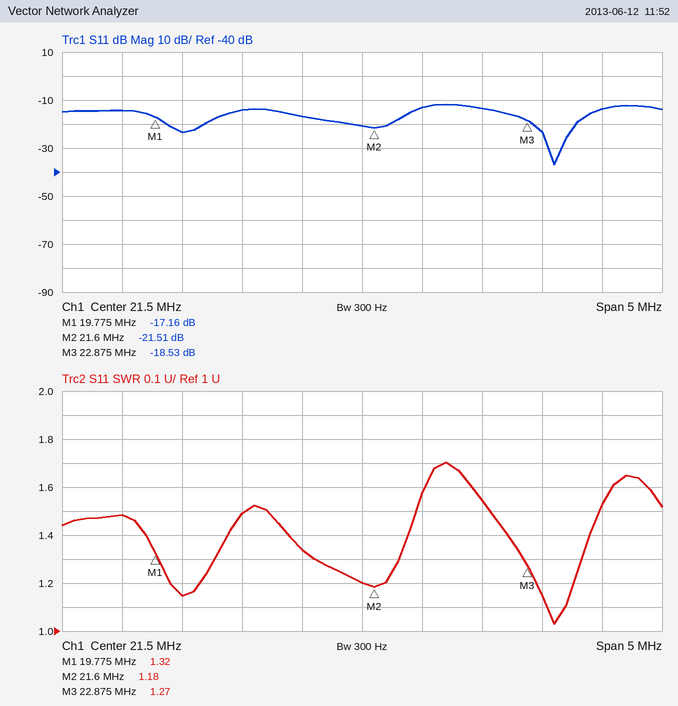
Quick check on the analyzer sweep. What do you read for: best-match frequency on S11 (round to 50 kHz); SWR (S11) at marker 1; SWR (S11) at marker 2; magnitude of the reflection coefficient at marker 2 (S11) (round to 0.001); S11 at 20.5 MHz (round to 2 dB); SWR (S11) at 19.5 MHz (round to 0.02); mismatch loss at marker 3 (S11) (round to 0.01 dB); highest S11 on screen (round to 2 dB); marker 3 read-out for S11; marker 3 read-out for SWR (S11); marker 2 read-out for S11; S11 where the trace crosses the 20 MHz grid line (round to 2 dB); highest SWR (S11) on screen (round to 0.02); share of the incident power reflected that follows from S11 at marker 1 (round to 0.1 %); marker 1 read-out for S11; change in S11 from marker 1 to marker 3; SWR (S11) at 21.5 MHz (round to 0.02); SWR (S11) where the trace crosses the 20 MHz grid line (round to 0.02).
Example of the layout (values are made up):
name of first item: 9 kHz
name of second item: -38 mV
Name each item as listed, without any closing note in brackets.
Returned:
best-match frequency on S11: 23.10 MHz
SWR (S11) at marker 1: 1.32
SWR (S11) at marker 2: 1.18
magnitude of the reflection coefficient at marker 2 (S11): 0.084
S11 at 20.5 MHz: -14 dB
SWR (S11) at 19.5 MHz: 1.48
mismatch loss at marker 3 (S11): 0.06 dB
highest S11 on screen: -12 dB
marker 3 read-out for S11: -18.53 dB
marker 3 read-out for SWR: 1.27
marker 2 read-out for S11: -21.51 dB
S11 where the trace crosses the 20 MHz grid line: -24 dB
highest SWR (S11) on screen: 1.70
share of the incident power reflected that follows from S11 at marker 1: 1.9 %
marker 1 read-out for S11: -17.16 dB
change in S11 from marker 1 to marker 3: -1.37 dB
SWR (S11) at 21.5 MHz: 1.20
SWR (S11) where the trace crosses the 20 MHz grid line: 1.14
